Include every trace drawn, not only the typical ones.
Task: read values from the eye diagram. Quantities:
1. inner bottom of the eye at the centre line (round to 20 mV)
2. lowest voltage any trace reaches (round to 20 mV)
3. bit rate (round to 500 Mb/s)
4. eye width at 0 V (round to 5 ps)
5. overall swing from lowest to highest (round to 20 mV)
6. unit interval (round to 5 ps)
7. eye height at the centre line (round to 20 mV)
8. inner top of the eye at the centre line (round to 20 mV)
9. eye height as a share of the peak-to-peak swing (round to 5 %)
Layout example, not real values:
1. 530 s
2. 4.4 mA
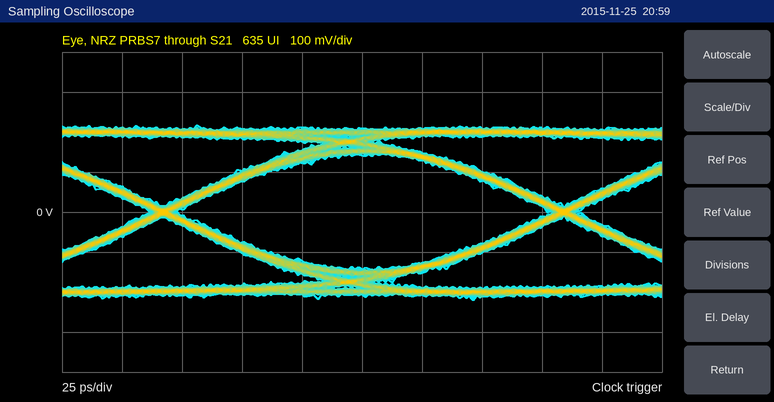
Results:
1. -140 mV
2. -220 mV
3. 6.0 Gb/s
4. 155 ps
5. 440 mV
6. 165 ps
7. 280 mV
8. 140 mV
9. 65 %
